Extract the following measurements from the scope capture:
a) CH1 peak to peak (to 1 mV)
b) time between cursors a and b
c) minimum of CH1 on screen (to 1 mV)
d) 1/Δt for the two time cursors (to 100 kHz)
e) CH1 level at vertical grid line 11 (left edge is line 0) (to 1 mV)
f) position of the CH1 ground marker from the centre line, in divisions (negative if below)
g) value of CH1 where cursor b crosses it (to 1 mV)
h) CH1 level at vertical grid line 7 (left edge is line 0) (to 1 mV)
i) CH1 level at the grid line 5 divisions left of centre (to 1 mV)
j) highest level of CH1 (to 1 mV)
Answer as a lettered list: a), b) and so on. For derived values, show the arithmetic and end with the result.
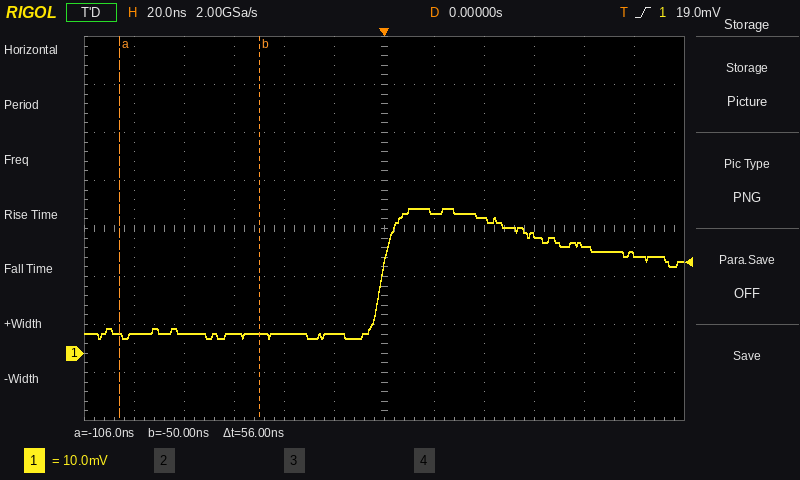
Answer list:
a) 30 mV − (3 mV) = 27 mV
b) 56 ns
c) 3 mV
d) 1 / 56 ns ≈ 17.9 MHz
e) 21 mV
f) -2.6 div
g) 4 mV
h) 29 mV
i) 4 mV
j) 30 mV
